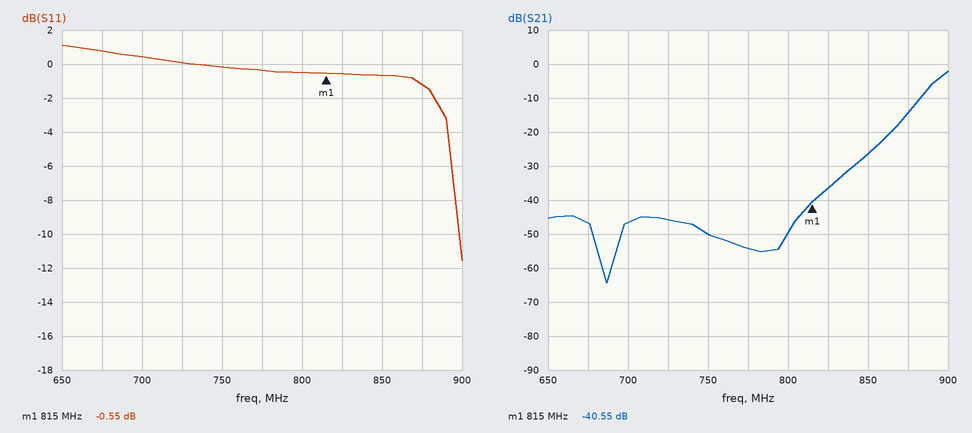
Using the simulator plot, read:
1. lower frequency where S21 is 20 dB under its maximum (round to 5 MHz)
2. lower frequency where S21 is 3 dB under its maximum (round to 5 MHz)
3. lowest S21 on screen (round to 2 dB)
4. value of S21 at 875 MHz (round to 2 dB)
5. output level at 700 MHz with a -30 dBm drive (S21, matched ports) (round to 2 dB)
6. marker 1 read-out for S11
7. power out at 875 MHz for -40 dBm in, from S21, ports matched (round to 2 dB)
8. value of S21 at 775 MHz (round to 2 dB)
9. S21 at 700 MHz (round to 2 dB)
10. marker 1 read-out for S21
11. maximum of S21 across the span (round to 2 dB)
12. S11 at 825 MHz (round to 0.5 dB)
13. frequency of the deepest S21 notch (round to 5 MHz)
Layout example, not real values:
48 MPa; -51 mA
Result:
860 MHz; 890 MHz; -64 dB; -14 dB; -76 dBm; -0.55 dB; -54 dBm; -54 dB; -46 dB; -40.55 dB; -2 dB; -0.5 dB; 685 MHz
